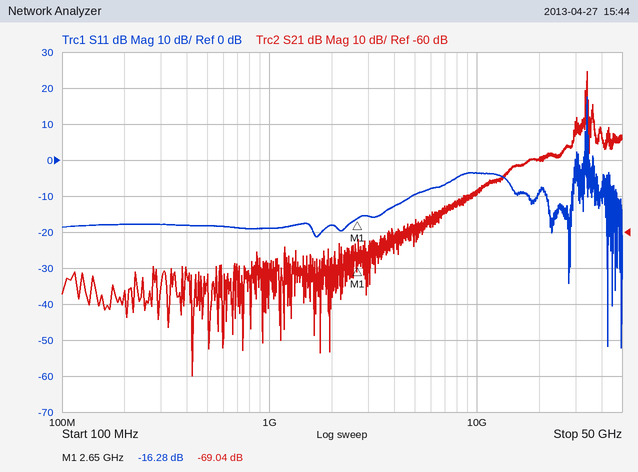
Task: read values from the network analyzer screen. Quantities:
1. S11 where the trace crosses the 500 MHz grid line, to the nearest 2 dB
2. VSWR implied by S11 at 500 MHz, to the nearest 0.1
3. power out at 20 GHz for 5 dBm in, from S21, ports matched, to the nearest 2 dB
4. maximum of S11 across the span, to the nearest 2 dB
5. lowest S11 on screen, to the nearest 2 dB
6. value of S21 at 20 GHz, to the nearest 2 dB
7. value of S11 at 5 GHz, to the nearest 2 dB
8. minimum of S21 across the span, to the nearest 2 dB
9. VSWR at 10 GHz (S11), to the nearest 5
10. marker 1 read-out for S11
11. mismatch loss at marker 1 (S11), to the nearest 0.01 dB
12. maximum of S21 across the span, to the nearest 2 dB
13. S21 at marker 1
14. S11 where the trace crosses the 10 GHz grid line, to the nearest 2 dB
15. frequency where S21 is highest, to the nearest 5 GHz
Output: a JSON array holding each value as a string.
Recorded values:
["-18 dB", "1.3", "-34 dBm", "18 dB", "-52 dB", "-40 dB", "-10 dB", "-100 dB", "5", "-16.28 dB", "0.10 dB", "-16 dB", "-69.04 dB", "-4 dB", "35 GHz"]
